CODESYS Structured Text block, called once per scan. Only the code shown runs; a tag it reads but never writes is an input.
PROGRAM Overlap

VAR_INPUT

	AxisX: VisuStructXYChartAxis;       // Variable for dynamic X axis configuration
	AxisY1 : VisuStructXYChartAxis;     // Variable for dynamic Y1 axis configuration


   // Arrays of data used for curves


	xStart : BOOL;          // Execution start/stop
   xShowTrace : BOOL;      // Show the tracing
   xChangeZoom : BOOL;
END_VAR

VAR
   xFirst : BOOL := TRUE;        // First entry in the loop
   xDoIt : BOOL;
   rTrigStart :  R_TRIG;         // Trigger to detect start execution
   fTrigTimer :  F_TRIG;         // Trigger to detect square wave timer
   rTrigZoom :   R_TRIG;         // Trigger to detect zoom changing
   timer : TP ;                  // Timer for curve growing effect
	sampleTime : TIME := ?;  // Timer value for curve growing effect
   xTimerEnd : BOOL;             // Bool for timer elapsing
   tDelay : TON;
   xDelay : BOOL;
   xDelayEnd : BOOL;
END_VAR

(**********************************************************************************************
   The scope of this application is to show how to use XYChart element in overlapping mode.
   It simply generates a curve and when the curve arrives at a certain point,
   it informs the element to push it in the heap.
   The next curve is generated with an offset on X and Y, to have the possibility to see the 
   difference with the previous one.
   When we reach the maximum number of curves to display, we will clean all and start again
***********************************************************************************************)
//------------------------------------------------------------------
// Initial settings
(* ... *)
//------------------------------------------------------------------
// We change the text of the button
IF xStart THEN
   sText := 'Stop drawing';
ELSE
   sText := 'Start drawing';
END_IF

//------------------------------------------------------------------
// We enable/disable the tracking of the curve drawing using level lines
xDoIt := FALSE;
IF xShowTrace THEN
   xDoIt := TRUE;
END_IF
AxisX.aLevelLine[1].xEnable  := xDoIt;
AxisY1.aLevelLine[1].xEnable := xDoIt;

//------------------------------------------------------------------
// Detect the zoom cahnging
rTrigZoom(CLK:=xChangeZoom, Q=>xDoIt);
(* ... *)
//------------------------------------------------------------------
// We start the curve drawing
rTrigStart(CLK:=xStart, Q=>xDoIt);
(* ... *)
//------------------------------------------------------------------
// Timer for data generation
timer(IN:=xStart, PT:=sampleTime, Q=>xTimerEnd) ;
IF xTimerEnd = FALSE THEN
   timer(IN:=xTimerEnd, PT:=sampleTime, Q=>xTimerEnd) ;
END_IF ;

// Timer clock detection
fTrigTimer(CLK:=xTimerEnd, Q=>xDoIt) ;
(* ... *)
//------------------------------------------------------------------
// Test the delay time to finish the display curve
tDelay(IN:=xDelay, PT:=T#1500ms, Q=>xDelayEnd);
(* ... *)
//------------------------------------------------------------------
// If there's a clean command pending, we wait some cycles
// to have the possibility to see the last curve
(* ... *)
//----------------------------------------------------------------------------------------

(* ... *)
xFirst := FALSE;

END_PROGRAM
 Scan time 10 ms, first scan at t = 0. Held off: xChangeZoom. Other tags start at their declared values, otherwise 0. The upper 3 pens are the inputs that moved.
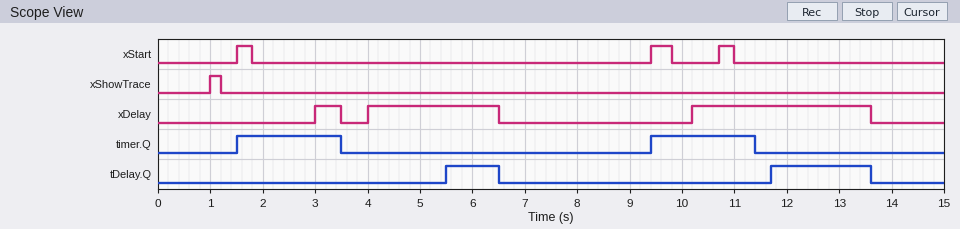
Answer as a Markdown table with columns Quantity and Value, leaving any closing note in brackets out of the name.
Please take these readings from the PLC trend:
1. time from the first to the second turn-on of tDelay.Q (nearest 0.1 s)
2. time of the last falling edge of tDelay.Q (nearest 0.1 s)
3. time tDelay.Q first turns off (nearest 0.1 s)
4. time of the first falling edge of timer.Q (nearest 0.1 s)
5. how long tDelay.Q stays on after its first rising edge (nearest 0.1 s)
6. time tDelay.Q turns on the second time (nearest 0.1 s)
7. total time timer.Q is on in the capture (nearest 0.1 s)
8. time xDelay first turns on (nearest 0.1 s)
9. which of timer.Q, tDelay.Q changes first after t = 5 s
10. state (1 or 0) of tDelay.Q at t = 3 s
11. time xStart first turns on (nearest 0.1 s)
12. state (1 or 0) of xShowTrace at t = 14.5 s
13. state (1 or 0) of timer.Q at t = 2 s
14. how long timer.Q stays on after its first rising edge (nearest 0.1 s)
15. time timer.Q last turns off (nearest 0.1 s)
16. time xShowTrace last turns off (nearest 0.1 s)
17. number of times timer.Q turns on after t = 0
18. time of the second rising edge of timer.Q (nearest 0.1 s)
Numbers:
| Quantity | Value |
|---|---|
| time from the first to the second turn-on of tDelay.Q | 6.2 s |
| time of the last falling edge of tDelay.Q | 13.6 s |
| time tDelay.Q first turns off | 6.5 s |
| time of the first falling edge of timer.Q | 3.5 s |
| how long tDelay.Q stays on after its first rising edge | 1.0 s |
| time tDelay.Q turns on the second time | 11.7 s |
| total time timer.Q is on in the capture | 4.0 s |
| time xDelay first turns on | 3.0 s |
| which of timer.Q, tDelay.Q changes first after t = 5 s | tDelay.Q |
| state (1 or 0) of tDelay.Q at t = 3 s | 0 |
| time xStart first turns on | 1.5 s |
| state (1 or 0) of xShowTrace at t = 14.5 s | 0 |
| state (1 or 0) of timer.Q at t = 2 s | 1 |
| how long timer.Q stays on after its first rising edge | 2.0 s |
| time timer.Q last turns off | 11.4 s |
| time xShowTrace last turns off | 1.2 s |
| number of times timer.Q turns on after t = 0 | 2 |
| time of the second rising edge of timer.Q | 9.4 s |
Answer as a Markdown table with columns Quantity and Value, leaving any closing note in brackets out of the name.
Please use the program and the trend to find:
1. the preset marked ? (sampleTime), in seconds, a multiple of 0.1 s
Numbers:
| Quantity | Value |
|---|---|
| the preset marked ? (sampleTime), in seconds, a multiple of 0.1 s | 2.0 s |
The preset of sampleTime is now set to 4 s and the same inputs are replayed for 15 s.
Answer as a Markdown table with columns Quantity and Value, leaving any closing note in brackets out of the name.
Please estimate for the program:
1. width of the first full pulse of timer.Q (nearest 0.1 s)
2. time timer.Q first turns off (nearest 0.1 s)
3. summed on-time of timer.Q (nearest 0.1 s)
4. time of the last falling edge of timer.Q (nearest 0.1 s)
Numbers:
| Quantity | Value |
|---|---|
| width of the first full pulse of timer.Q | 4.0 s |
| time timer.Q first turns off | 5.5 s |
| summed on-time of timer.Q | 8.0 s |
| time of the last falling edge of timer.Q | 13.4 s |
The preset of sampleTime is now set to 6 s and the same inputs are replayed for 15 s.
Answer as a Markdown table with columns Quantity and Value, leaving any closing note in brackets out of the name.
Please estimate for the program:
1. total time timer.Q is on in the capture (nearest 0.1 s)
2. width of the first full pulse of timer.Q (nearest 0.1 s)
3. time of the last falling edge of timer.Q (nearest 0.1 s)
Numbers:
| Quantity | Value |
|---|---|
| total time timer.Q is on in the capture | 11.6 s |
| width of the first full pulse of timer.Q | 6.0 s |
| time of the last falling edge of timer.Q | 7.5 s |
